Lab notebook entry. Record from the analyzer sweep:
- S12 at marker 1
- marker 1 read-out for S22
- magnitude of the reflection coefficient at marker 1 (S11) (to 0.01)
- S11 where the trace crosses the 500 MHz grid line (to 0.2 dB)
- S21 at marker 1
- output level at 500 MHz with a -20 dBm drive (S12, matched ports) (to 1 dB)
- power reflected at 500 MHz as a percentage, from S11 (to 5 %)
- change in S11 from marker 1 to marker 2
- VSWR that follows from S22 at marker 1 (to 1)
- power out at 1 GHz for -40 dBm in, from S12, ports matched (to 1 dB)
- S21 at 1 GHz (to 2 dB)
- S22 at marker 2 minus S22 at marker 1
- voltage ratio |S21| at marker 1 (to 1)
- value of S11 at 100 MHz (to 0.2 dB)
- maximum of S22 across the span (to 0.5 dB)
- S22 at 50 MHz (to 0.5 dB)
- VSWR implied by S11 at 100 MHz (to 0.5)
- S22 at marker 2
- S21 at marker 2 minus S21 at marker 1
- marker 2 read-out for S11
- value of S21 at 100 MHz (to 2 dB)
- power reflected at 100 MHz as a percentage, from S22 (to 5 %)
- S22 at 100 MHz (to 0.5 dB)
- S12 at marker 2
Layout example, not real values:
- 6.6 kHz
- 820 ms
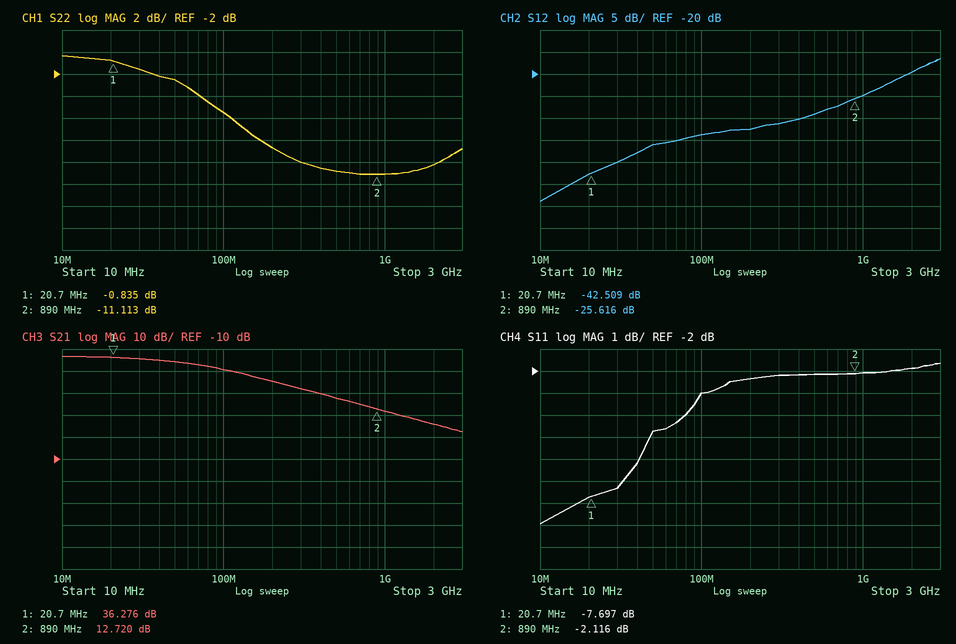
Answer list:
- -42.509 dB
- -0.835 dB
- 0.41
- -2.2 dB
- 36.276 dB
- -49 dBm
- 60 %
- 5.581 dB
- 21
- -65 dBm
- 12 dB
- -10.278 dB
- 65
- -3.0 dB
- -0.5 dB
- -2.5 dB
- 6.0
- -11.113 dB
- -23.556 dB
- -2.116 dB
- 30 dB
- 30 %
- -5.5 dB
- -25.616 dB
